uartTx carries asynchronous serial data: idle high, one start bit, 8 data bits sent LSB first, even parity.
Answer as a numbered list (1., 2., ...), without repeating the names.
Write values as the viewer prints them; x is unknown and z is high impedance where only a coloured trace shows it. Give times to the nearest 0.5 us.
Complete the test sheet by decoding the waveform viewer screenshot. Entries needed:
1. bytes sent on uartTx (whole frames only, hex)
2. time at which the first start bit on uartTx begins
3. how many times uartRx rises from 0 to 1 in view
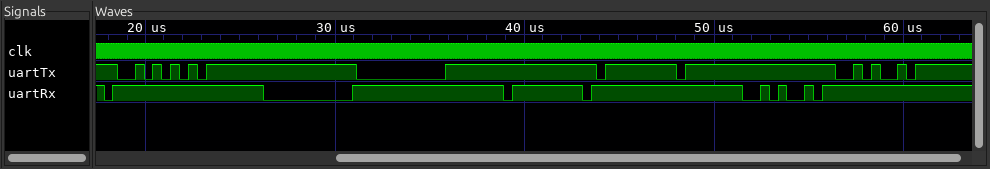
1. AA, 00, FF, 4A
2. 18.5 us
3. 8
